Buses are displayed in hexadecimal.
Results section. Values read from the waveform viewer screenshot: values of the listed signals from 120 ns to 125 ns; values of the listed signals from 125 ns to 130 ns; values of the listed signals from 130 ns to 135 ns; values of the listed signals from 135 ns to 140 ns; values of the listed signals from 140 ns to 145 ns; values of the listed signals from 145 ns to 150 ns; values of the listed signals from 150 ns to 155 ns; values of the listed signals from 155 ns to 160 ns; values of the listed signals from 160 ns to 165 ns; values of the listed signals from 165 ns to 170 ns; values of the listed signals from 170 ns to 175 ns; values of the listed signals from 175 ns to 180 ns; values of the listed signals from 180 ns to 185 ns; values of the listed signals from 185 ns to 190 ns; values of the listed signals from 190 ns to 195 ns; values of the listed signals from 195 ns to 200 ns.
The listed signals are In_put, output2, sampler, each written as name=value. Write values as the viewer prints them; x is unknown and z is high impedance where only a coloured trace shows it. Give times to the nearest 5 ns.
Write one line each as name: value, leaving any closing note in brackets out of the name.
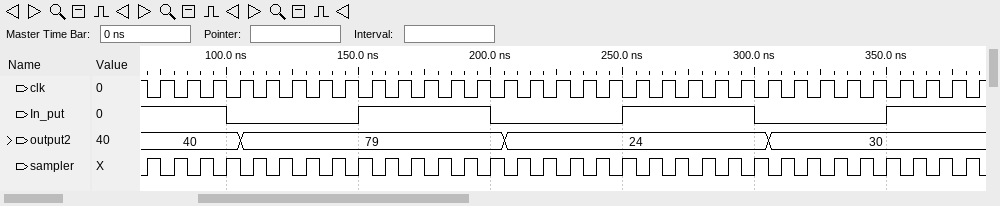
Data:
values of the listed signals from 120 ns to 125 ns: In_put=0, output2=79, sampler=1
values of the listed signals from 125 ns to 130 ns: In_put=0, output2=79, sampler=0
values of the listed signals from 130 ns to 135 ns: In_put=0, output2=79, sampler=1
values of the listed signals from 135 ns to 140 ns: In_put=0, output2=79, sampler=0
values of the listed signals from 140 ns to 145 ns: In_put=0, output2=79, sampler=1
values of the listed signals from 145 ns to 150 ns: In_put=0, output2=79, sampler=0
values of the listed signals from 150 ns to 155 ns: In_put=1, output2=79, sampler=1
values of the listed signals from 155 ns to 160 ns: In_put=1, output2=79, sampler=0
values of the listed signals from 160 ns to 165 ns: In_put=1, output2=79, sampler=1
values of the listed signals from 165 ns to 170 ns: In_put=1, output2=79, sampler=0
values of the listed signals from 170 ns to 175 ns: In_put=1, output2=79, sampler=1
values of the listed signals from 175 ns to 180 ns: In_put=1, output2=79, sampler=0
values of the listed signals from 180 ns to 185 ns: In_put=1, output2=79, sampler=1
values of the listed signals from 185 ns to 190 ns: In_put=1, output2=79, sampler=0
values of the listed signals from 190 ns to 195 ns: In_put=1, output2=79, sampler=1
values of the listed signals from 195 ns to 200 ns: In_put=1, output2=79, sampler=0
